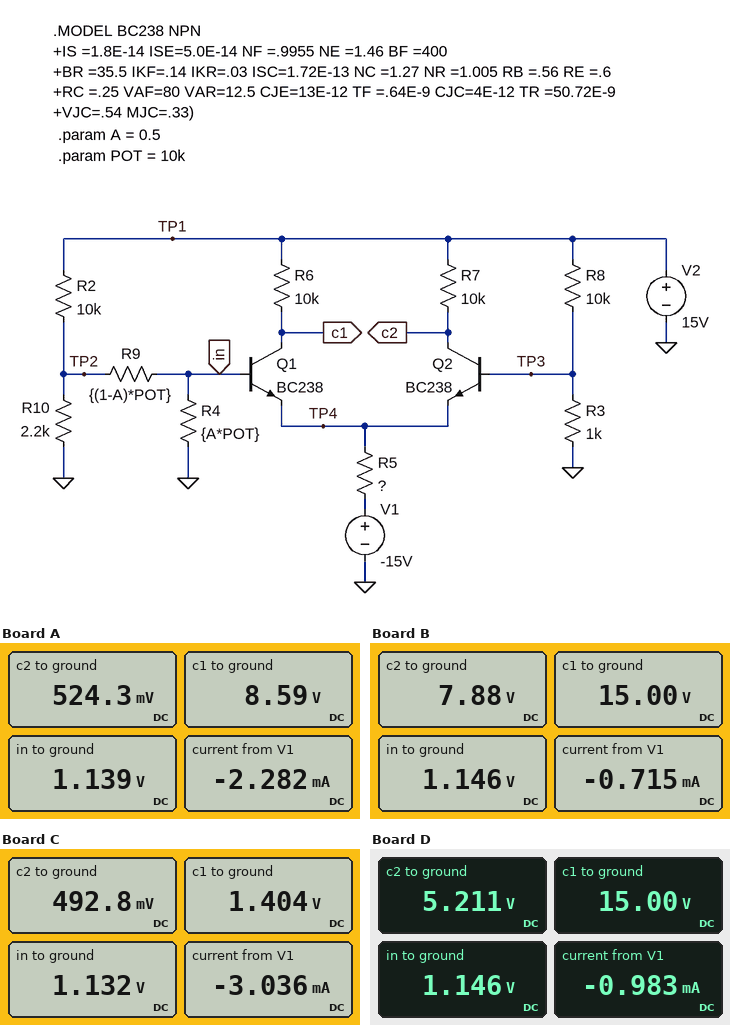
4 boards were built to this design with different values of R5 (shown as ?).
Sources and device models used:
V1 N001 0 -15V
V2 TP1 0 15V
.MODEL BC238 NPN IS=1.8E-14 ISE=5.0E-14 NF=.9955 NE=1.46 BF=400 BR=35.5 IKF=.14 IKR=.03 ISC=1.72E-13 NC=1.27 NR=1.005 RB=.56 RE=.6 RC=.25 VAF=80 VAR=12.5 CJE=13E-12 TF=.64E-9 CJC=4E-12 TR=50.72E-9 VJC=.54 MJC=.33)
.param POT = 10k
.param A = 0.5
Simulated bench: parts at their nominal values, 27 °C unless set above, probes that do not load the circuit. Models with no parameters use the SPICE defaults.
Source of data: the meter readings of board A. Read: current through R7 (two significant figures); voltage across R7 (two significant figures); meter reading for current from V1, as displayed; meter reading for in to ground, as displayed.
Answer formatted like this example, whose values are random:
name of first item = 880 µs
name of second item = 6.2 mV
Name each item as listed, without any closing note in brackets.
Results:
current through R7 = 1.4 mA
voltage across R7 = 14 V
meter reading for current from V1, as displayed = -2.282 mA
meter reading for in to ground, as displayed = 1.139 V
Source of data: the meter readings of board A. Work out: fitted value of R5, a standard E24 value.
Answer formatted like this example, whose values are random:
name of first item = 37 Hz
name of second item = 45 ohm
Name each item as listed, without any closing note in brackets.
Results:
fitted value of R5, a standard E24 value = 6.8 kΩ
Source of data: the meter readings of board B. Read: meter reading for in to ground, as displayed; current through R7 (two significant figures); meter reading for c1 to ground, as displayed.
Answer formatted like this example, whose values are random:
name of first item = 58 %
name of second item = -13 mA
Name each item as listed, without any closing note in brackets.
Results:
meter reading for in to ground, as displayed = 1.146 V
current through R7 = 710 µA
meter reading for c1 to ground, as displayed = 15.00 V
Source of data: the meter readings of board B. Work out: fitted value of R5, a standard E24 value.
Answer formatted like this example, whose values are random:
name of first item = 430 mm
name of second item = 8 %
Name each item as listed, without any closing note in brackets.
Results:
fitted value of R5, a standard E24 value = 22 kΩ
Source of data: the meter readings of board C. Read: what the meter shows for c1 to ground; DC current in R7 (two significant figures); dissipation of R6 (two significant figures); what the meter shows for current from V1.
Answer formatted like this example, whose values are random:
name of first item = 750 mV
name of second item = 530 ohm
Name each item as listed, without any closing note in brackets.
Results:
what the meter shows for c1 to ground = 1.404 V
DC current in R7 = 1.5 mA
dissipation of R6 = 18 mW
what the meter shows for current from V1 = -3.036 mA
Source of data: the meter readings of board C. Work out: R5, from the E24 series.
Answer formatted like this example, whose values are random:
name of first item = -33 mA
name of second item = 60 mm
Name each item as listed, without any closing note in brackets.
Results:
R5, from the E24 series = 5.1 kΩ
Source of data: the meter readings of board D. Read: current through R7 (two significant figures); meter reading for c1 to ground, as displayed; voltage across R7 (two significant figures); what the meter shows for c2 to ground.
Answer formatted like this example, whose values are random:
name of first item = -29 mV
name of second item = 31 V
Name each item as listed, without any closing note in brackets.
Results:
current through R7 = 980 µA
meter reading for c1 to ground, as displayed = 15.00 V
voltage across R7 = 9.8 V
what the meter shows for c2 to ground = 5.211 V
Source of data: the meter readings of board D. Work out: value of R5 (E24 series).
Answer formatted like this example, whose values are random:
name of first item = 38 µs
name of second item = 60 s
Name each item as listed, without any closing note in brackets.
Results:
value of R5 = 16 kΩ
